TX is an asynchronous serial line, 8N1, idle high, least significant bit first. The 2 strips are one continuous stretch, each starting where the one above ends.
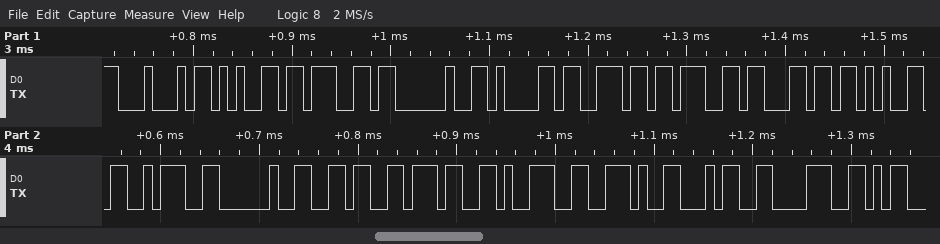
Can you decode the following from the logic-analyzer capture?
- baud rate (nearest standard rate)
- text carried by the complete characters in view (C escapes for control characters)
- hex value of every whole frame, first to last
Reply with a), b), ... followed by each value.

a) 115200 baud
b) "Deg angle: 679.48"
c) 44 65 67 20 61 6E 67 6C 65 3A 20 36 37 39 2E 34 38
